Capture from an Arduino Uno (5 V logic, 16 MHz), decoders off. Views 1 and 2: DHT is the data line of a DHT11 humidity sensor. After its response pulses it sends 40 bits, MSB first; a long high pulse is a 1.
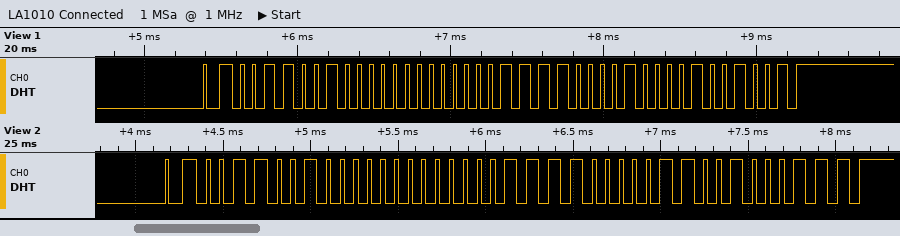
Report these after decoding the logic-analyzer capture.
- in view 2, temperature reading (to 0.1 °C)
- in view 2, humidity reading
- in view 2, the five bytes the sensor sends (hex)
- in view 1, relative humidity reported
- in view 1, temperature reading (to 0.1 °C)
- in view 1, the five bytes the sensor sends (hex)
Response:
15.6 °C
50 %
32 00 0F 06 47
50 %
15.8 °C
32 00 0F 08 49
